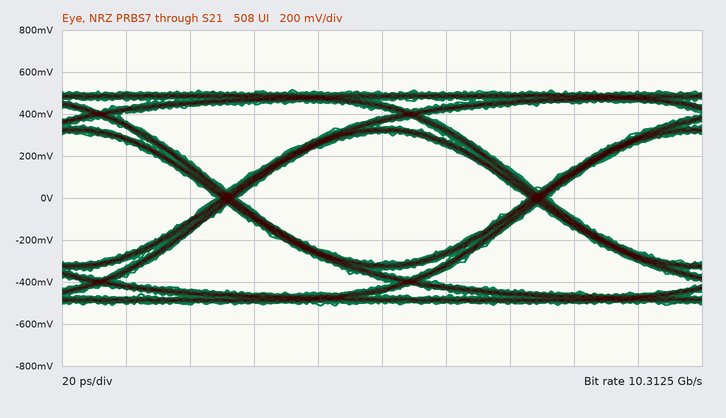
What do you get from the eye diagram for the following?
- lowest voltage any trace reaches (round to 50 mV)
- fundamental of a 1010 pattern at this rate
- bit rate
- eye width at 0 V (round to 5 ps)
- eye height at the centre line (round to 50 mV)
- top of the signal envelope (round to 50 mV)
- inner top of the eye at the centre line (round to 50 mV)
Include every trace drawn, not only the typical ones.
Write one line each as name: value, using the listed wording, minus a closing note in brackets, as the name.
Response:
lowest voltage any trace reaches: -500 mV
fundamental of a 1010 pattern at this rate: 5.15625 GHz
bit rate: 10.3125 Gb/s
eye width at 0 V: 90 ps
eye height at the centre line: 600 mV
top of the signal envelope: 500 mV
inner top of the eye at the centre line: 300 mV
